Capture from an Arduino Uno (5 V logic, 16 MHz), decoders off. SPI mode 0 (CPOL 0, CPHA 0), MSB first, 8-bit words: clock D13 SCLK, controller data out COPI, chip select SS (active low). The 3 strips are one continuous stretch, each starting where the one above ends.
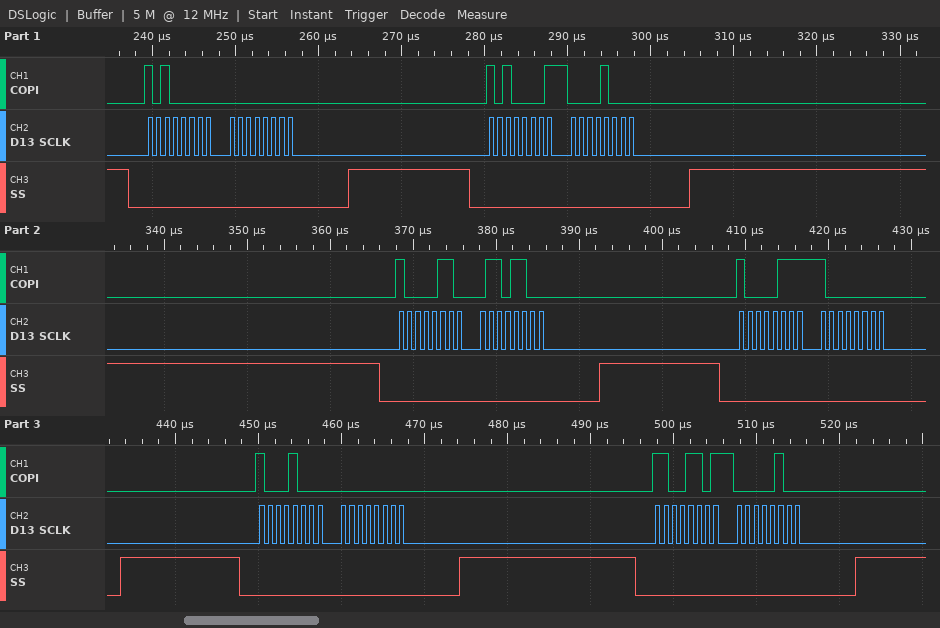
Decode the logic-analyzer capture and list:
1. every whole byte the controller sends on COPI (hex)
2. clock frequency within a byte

A0 00 A1 08 86 6C 87 80 88 00 CD 04
1 MHz
